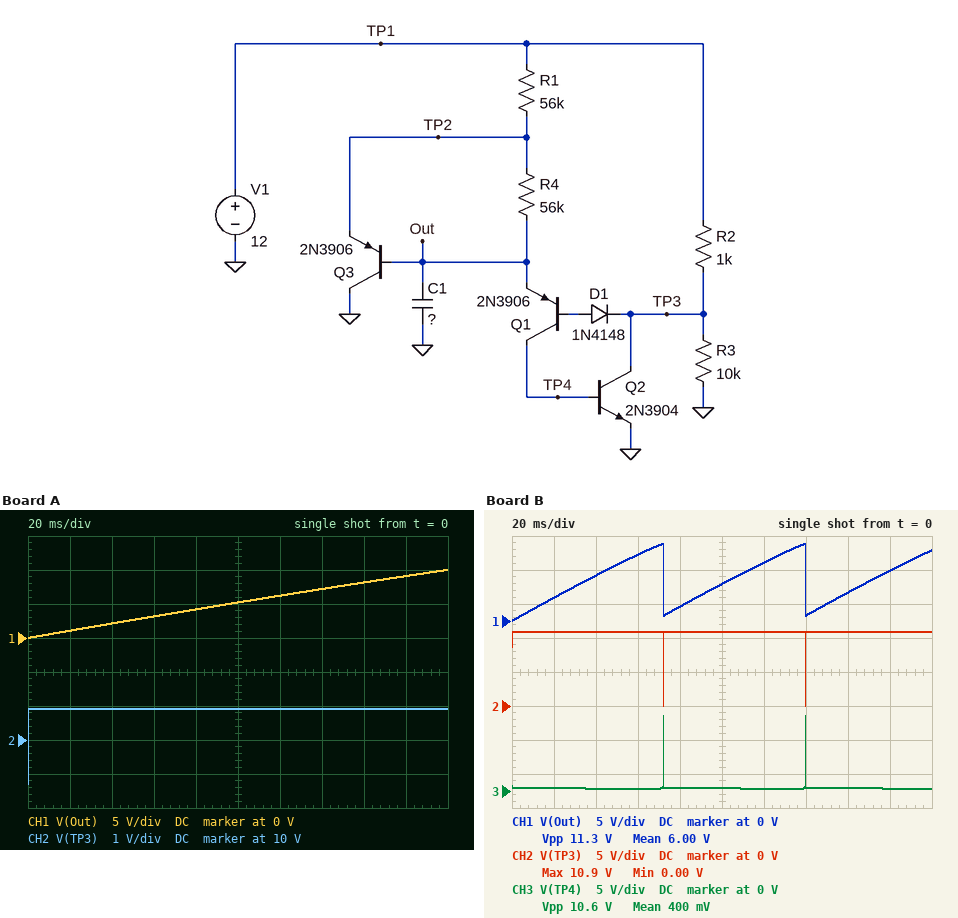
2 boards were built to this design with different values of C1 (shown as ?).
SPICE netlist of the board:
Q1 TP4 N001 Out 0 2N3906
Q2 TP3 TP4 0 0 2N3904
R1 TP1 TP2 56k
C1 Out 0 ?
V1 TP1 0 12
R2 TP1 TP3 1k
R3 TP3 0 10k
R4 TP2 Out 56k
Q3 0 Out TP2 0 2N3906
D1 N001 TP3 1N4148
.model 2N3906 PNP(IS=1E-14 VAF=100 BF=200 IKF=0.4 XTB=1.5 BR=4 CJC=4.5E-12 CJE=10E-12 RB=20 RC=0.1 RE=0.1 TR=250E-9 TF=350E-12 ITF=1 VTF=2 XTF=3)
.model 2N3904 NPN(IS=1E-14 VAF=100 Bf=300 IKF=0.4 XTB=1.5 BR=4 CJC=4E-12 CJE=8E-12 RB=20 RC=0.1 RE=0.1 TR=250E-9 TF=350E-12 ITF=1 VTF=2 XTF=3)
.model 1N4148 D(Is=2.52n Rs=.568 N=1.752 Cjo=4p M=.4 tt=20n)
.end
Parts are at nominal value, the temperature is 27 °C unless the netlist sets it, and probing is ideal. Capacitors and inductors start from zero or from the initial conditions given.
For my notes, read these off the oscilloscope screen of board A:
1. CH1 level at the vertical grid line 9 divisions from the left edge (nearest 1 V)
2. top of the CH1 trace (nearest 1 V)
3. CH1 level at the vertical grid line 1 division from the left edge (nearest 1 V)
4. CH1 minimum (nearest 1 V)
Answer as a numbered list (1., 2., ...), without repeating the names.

1. 9 V
2. 10 V
3. 1 V
4. 0 V
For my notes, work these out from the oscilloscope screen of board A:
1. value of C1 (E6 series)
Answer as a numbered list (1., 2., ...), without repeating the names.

1. 220 nF
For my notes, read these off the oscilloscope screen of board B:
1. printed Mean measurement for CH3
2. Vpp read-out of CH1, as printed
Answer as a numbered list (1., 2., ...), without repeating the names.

1. 400 mV
2. 11.3 V
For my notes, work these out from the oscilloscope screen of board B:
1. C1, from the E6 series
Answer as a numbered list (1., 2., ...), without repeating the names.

1. 68 nF
